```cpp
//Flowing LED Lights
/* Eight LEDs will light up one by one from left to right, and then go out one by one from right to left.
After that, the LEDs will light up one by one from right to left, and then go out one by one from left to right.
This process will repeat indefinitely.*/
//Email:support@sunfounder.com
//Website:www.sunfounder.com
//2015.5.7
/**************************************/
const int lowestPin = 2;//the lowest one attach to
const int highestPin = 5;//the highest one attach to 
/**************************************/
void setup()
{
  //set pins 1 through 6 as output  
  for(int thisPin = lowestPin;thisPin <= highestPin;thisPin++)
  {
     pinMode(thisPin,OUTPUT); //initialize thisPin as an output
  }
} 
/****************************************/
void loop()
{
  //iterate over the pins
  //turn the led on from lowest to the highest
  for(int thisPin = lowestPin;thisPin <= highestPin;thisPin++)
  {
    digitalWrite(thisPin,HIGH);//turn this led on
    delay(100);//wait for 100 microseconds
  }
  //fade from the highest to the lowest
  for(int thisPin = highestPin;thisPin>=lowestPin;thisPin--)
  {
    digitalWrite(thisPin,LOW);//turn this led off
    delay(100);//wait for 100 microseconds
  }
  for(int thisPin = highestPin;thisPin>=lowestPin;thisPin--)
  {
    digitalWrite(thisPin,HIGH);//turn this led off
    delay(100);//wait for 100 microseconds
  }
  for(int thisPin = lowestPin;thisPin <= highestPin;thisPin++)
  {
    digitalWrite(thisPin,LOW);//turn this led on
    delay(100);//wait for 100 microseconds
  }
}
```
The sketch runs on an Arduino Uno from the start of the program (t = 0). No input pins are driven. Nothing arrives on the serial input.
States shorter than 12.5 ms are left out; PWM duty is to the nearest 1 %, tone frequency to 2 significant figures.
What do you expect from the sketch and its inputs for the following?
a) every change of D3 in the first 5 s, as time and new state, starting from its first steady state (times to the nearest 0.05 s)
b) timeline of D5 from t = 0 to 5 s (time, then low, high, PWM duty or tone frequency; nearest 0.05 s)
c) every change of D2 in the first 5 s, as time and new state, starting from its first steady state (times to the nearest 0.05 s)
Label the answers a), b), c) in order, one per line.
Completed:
a) 0 s low; 0.1 s high; 0.6 s low; 1 s high; 1.3 s low; 1.7 s high; 2.2 s low; 2.6 s high; 2.9 s low; 3.3 s high; 3.8 s low; 4.2 s high; 4.5 s low; 4.9 s high
b) 0 s low; 0.3 s high; 0.4 s low; 0.8 s high; 1.5 s low; 1.9 s high; 2 s low; 2.4 s high; 3.1 s low; 3.5 s high; 3.6 s low; 4 s high; 4.7 s low
c) 0 s high; 0.7 s low; 1.1 s high; 1.2 s low; 1.6 s high; 2.3 s low; 2.7 s high; 2.8 s low; 3.2 s high; 3.9 s low; 4.3 s high; 4.4 s low; 4.8 s high
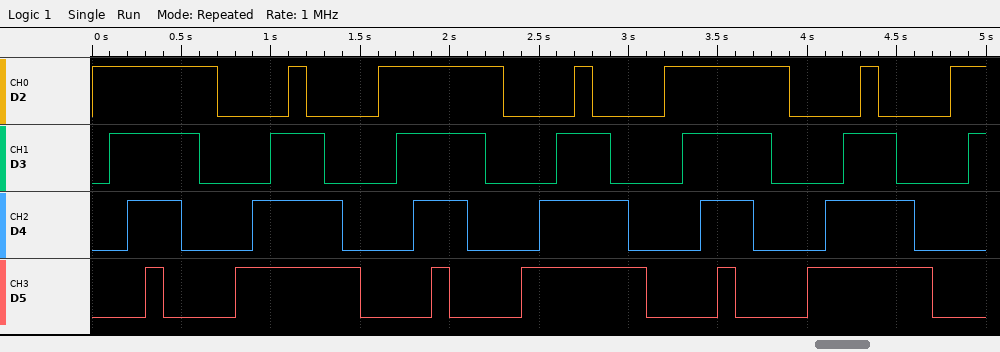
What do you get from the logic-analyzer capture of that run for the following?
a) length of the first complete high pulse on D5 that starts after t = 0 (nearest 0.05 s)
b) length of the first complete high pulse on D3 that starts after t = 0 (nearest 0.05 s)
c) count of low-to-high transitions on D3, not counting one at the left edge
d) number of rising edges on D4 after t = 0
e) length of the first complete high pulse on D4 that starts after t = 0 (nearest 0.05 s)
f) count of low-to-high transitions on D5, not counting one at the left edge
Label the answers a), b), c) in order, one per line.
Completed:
a) 0.10 s
b) 0.50 s
c) 7
d) 6
e) 0.30 s
f) 6
